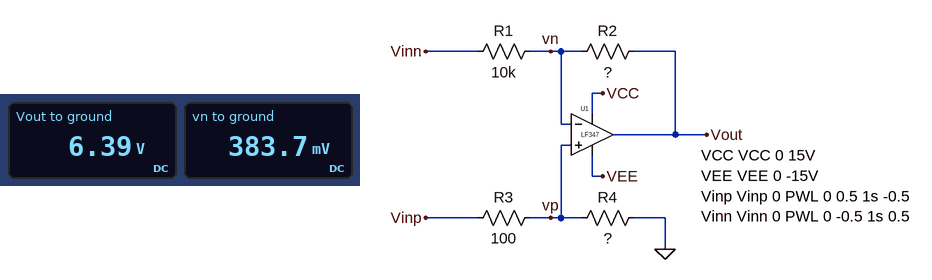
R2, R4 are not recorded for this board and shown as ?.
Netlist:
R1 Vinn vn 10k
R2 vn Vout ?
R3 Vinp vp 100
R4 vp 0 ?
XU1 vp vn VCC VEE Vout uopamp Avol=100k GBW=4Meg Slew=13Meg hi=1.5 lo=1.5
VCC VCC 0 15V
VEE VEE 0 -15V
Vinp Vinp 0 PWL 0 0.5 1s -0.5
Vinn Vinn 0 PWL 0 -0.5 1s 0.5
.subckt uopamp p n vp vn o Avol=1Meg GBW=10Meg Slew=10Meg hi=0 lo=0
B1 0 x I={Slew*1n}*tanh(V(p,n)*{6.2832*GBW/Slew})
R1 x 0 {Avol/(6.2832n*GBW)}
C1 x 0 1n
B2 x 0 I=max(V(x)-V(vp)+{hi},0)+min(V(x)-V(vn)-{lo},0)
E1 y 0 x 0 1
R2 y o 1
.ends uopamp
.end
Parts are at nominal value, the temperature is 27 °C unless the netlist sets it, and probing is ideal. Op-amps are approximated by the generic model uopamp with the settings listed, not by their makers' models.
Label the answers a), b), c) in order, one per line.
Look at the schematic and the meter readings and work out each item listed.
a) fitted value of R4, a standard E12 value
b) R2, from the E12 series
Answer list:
a) 330 Ω
b) 68 kΩ
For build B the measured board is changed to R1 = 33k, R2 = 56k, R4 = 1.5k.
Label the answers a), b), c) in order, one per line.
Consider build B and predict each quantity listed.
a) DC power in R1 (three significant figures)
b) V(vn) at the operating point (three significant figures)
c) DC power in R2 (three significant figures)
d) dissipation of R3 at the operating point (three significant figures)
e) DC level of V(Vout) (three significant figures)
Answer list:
a) 28.4 µW
b) 469 mV
c) 48.3 µW
d) 9.77 µW
e) 2.11 V
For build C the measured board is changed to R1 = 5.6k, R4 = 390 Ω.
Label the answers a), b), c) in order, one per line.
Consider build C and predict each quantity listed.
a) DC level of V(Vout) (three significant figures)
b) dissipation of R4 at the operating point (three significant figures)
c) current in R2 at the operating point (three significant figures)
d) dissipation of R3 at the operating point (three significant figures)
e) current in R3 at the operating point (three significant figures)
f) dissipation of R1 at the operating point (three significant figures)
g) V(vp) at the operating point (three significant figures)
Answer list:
a) 11.3 V
b) 406 µW
c) 160 µA
d) 104 µW
e) 1.02 mA
f) 144 µW
g) 398 mV
